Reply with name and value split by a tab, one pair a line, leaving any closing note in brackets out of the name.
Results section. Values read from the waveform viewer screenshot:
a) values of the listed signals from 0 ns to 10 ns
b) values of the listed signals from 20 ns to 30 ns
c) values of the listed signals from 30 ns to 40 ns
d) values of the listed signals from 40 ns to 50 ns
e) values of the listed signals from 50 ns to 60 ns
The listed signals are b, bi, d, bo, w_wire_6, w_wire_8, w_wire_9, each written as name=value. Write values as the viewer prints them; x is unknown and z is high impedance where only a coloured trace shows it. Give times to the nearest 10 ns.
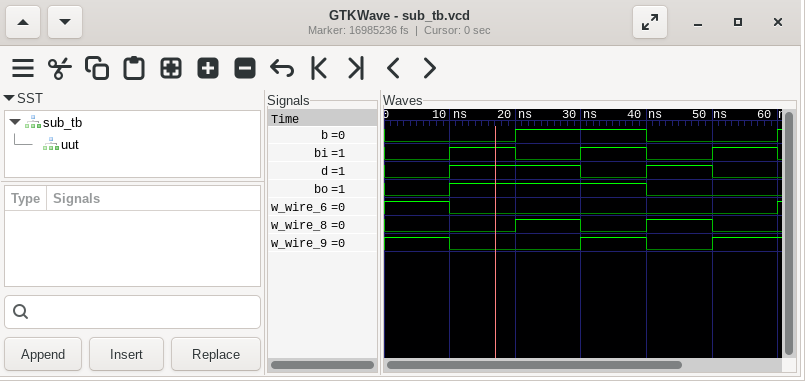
values of the listed signals from 0 ns to 10 ns	b=0, bi=0, d=0, bo=0, w_wire_6=1, w_wire_8=0, w_wire_9=1
values of the listed signals from 20 ns to 30 ns	b=1, bi=0, d=1, bo=1, w_wire_6=0, w_wire_8=1, w_wire_9=0
values of the listed signals from 30 ns to 40 ns	b=1, bi=1, d=0, bo=1, w_wire_6=0, w_wire_8=0, w_wire_9=1
values of the listed signals from 40 ns to 50 ns	b=0, bi=0, d=1, bo=0, w_wire_6=0, w_wire_8=1, w_wire_9=0
values of the listed signals from 50 ns to 60 ns	b=0, bi=1, d=0, bo=0, w_wire_6=0, w_wire_8=0, w_wire_9=1
